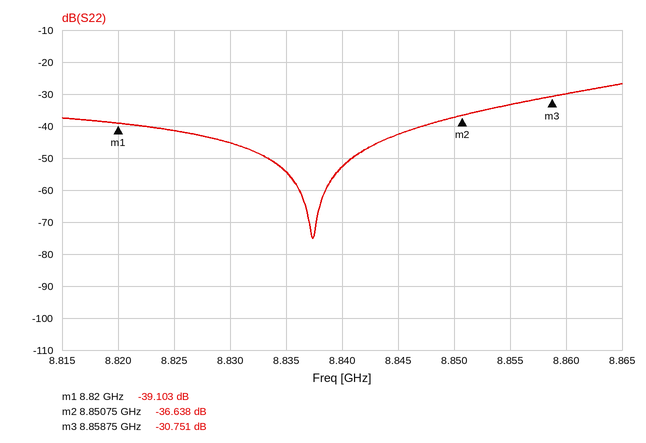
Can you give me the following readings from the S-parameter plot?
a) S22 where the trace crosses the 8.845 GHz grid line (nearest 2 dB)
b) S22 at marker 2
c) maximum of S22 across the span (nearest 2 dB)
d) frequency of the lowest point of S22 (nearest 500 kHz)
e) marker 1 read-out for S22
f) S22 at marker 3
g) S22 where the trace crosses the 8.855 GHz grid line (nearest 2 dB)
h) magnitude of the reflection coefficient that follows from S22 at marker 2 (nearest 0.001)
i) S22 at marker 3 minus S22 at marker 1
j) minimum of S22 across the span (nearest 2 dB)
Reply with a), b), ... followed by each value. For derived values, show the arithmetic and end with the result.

a) -42 dB
b) -36.638 dB
c) -26 dB
d) 8.8375 GHz
e) -39.103 dB
f) -30.751 dB
g) -34 dB
h) 10^(-36.638/20) ≈ 0.015
i) -30.751 − (-39.103) = 8.352 dB
j) -76 dB
